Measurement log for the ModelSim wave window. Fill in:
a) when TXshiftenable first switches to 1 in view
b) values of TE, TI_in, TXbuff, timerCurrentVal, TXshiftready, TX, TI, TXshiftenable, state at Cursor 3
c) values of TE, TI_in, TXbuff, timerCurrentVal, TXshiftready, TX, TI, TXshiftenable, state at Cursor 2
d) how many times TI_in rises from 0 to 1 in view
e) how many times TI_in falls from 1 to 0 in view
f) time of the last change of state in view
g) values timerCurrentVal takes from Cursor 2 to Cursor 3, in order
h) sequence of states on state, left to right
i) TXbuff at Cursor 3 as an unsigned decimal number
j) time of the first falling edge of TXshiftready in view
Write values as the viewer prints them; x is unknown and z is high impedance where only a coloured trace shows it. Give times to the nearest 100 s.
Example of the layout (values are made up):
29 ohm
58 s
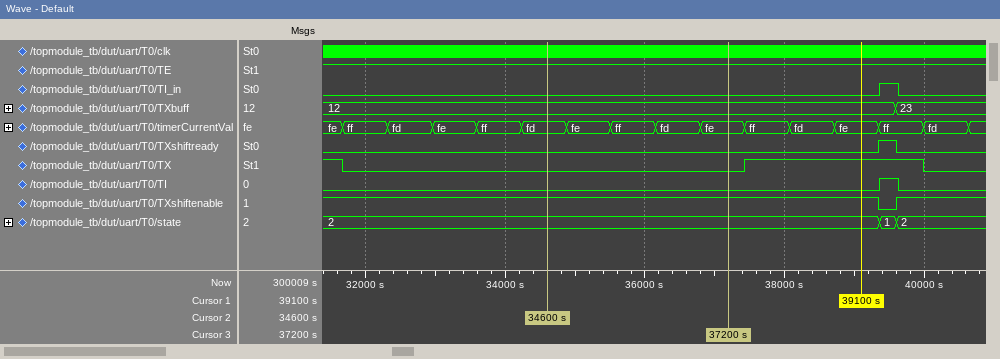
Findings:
39600 s
TE=1, TI_in=0, TXbuff=12, timerCurrentVal=fe, TXshiftready=0, TX=0, TI=0, TXshiftenable=1, state=2
TE=1, TI_in=0, TXbuff=12, timerCurrentVal=fd, TXshiftready=0, TX=0, TI=0, TXshiftenable=1, state=2
1
1
39600 s
fd, fe, ff, fd, fe
2, 1, 2
18
39600 s
